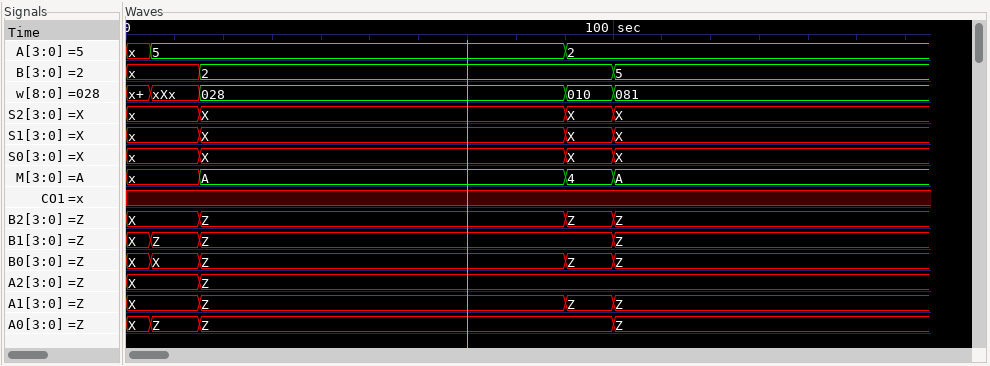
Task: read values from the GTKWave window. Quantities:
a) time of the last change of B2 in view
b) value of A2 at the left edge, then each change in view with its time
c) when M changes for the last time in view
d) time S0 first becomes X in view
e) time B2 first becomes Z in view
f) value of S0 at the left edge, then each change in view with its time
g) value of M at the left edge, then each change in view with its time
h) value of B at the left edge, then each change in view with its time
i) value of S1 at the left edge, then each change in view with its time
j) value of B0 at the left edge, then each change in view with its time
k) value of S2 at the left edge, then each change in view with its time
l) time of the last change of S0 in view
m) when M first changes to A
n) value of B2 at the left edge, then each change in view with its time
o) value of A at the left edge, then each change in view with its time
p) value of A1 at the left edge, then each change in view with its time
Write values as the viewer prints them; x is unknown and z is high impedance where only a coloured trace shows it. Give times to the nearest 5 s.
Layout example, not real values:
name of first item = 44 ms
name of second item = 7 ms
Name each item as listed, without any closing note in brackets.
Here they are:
time of the last change of B2 in view = 100 s
value of A2 at the left edge, then each change in view with its time = X, Z at 15 s
when M changes for the last time in view = 100 s
time S0 first becomes X in view = 15 s
time B2 first becomes Z in view = 15 s
value of S0 at the left edge, then each change in view with its time = x, X at 15 s, X at 90 s, X at 100 s
value of M at the left edge, then each change in view with its time = x, A at 15 s, 4 at 90 s, A at 100 s
value of B at the left edge, then each change in view with its time = x, 2 at 15 s, 5 at 100 s
value of S1 at the left edge, then each change in view with its time = x, X at 15 s, X at 90 s, X at 100 s
value of B0 at the left edge, then each change in view with its time = X, X at 5 s, Z at 15 s, Z at 90 s, Z at 100 s
value of S2 at the left edge, then each change in view with its time = x, X at 15 s, X at 90 s, X at 100 s
time of the last change of S0 in view = 100 s
when M first changes to A = 15 s
value of B2 at the left edge, then each change in view with its time = X, Z at 15 s, Z at 90 s, Z at 100 s
value of A at the left edge, then each change in view with its time = x, 5 at 5 s, 2 at 90 s
value of A1 at the left edge, then each change in view with its time = X, Z at 15 s, Z at 90 s, Z at 100 s
